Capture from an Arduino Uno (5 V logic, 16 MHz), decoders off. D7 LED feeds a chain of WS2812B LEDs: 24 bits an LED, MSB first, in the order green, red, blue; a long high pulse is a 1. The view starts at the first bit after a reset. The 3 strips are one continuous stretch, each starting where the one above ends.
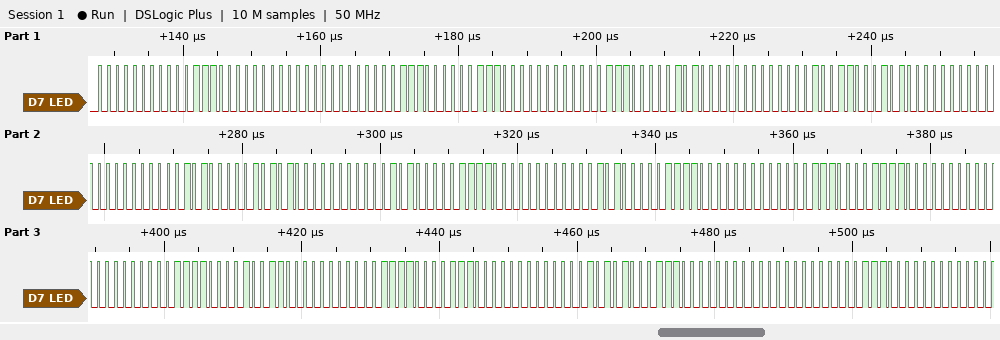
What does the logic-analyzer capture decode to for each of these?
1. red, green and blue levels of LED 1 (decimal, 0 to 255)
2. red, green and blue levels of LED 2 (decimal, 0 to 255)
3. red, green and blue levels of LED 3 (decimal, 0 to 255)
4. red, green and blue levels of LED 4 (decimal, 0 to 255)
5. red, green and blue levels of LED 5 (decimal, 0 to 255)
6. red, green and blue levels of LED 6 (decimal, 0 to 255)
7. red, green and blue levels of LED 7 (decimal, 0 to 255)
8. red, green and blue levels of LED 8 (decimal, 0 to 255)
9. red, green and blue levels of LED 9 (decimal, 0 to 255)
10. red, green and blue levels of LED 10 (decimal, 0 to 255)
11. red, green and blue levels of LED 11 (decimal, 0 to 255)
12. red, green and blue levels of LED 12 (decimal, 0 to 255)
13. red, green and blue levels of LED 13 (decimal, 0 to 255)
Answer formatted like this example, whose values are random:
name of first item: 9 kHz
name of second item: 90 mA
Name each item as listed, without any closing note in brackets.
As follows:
red, green and blue levels of LED 1: 28, 0, 0
red, green and blue levels of LED 2: 28, 0, 14
red, green and blue levels of LED 3: 28, 0, 20
red, green and blue levels of LED 4: 19, 0, 20
red, green and blue levels of LED 5: 0, 0, 20
red, green and blue levels of LED 6: 0, 21, 20
red, green and blue levels of LED 7: 0, 30, 20
red, green and blue levels of LED 8: 0, 30, 14
red, green and blue levels of LED 9: 0, 30, 0
red, green and blue levels of LED 10: 19, 30, 0
red, green and blue levels of LED 11: 28, 30, 0
red, green and blue levels of LED 12: 28, 21, 0
red, green and blue levels of LED 13: 28, 0, 0
